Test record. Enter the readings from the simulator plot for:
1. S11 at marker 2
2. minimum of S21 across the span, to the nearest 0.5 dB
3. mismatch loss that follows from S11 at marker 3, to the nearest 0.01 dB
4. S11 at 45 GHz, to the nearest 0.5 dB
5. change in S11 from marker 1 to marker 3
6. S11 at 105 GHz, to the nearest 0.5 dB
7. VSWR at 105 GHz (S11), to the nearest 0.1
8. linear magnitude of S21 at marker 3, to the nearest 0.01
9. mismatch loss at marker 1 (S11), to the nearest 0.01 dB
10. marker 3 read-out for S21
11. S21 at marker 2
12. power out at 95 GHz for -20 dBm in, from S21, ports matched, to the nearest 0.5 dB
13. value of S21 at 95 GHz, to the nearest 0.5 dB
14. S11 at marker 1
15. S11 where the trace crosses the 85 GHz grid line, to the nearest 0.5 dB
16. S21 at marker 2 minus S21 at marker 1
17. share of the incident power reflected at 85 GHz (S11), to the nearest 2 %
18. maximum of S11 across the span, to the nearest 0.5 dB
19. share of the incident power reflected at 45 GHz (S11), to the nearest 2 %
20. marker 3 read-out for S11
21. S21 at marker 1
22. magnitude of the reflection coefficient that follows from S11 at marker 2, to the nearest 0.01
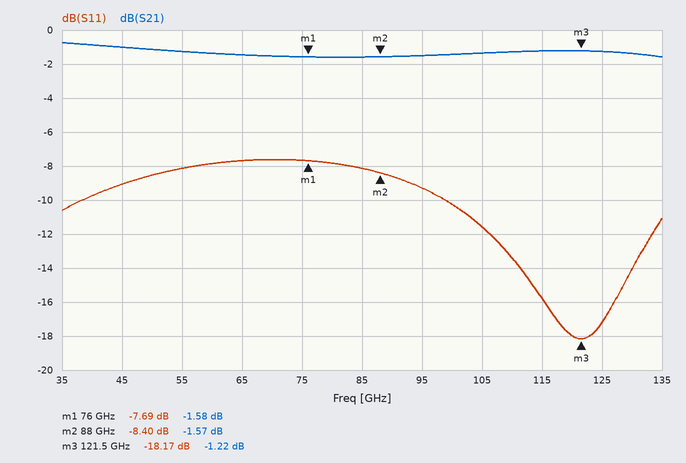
-8.40 dB
-1.5 dB
0.07 dB
-9.0 dB
-10.48 dB
-11.5 dB
1.7
0.87
0.81 dB
-1.22 dB
-1.57 dB
-21.5 dBm
-1.5 dB
-7.69 dB
-8.0 dB
0.01 dB
16 %
-7.5 dB
12 %
-18.17 dB
-1.58 dB
0.38
